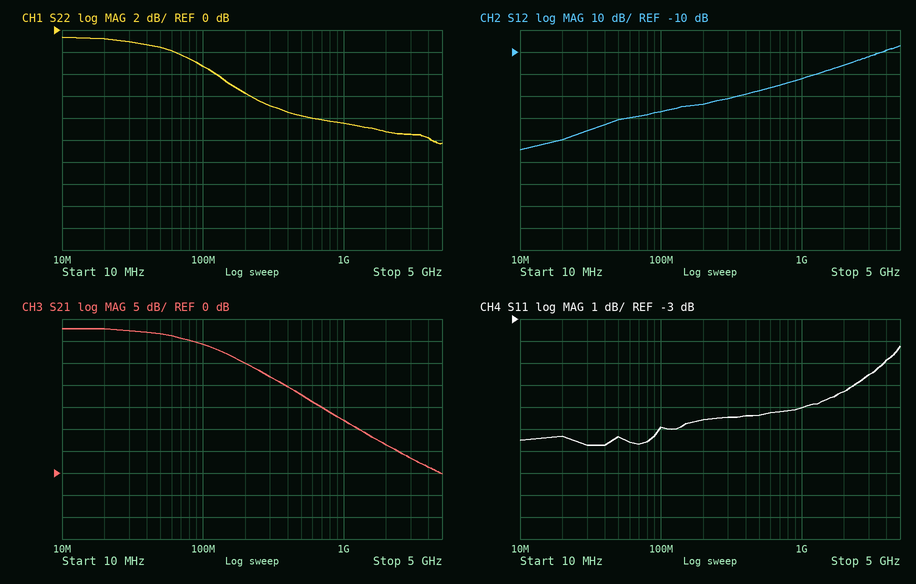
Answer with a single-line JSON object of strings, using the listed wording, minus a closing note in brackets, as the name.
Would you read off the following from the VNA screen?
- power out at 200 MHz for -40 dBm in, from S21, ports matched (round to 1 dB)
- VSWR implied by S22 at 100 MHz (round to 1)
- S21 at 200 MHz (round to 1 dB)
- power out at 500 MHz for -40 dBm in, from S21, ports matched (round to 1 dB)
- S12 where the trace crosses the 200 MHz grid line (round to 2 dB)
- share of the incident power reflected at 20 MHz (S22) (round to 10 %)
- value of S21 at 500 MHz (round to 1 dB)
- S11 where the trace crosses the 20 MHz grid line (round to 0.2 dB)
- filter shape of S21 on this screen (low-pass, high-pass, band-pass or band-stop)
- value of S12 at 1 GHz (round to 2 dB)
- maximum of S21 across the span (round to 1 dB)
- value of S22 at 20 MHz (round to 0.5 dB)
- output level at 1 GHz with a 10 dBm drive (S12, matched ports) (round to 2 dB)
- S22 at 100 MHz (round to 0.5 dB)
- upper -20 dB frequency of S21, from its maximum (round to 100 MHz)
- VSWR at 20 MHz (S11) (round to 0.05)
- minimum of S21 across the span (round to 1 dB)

{"power out at 200 MHz for -40 dBm in, from S21, ports matched": "-15 dBm", "VSWR implied by S22 at 100 MHz": "5", "S21 at 200 MHz": "25 dB", "power out at 500 MHz for -40 dBm in, from S21, ports matched": "-22 dBm", "S12 where the trace crosses the 200 MHz grid line": "-34 dB", "share of the incident power reflected at 20 MHz (S22)": "80 %", "value of S21 at 500 MHz": "18 dB", "S11 where the trace crosses the 20 MHz grid line": "-8.4 dB", "filter shape of S21 on this screen": "low-pass", "value of S12 at 1 GHz": "-22 dB", "maximum of S21 across the span": "33 dB", "value of S22 at 20 MHz": "-1.0 dB", "output level at 1 GHz with a 10 dBm drive (S12, matched ports)": "-12 dBm", "S22 at 100 MHz": "-3.5 dB", "upper -20 dB frequency of S21, from its maximum": "900 MHz", "VSWR at 20 MHz (S11)": "2.25", "minimum of S21 across the span": "0 dB"}
